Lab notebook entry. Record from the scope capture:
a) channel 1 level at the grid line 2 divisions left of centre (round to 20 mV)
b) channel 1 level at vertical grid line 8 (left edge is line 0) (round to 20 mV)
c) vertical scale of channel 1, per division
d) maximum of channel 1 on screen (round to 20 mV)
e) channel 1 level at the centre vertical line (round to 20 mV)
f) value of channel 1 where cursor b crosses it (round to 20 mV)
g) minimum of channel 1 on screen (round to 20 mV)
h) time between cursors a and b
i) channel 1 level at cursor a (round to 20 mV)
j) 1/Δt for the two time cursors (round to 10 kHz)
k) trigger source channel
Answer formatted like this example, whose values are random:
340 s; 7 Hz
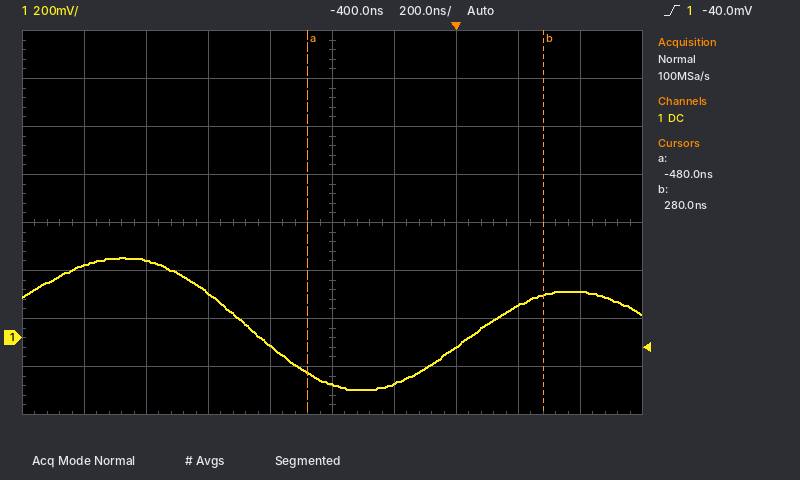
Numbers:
180 mV; 140 mV; 200 mV; 340 mV; -200 mV; 180 mV; -220 mV; 760 ns; -140 mV; 1.32 MHz; channel 1
